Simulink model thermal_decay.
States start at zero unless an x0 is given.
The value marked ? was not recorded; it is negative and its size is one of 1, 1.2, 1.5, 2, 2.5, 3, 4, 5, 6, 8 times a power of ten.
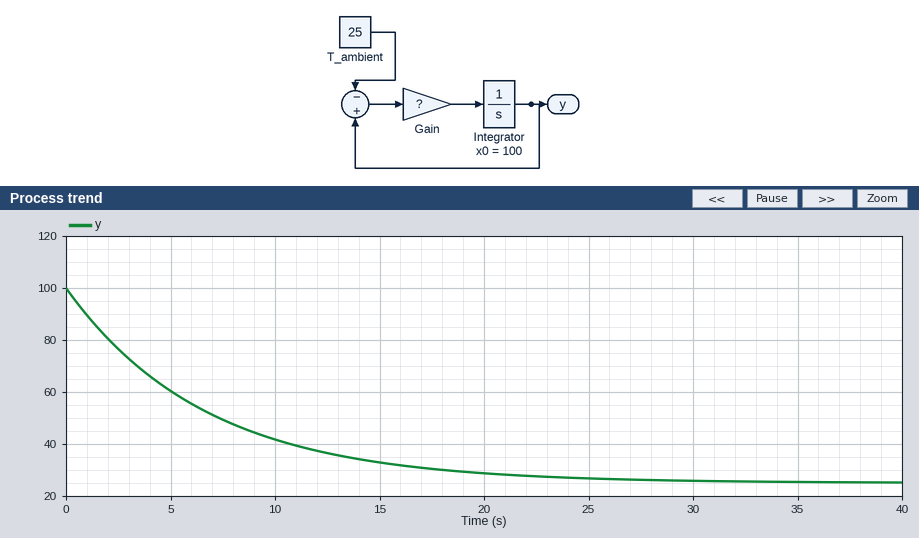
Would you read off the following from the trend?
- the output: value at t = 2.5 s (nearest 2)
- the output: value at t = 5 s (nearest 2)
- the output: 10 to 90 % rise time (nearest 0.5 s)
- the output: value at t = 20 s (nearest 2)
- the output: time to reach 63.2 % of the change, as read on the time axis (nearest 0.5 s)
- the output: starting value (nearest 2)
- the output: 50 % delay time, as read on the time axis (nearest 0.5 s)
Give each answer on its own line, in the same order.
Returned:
76
60
14.5 s
28
6.5 s
100
4.5 s
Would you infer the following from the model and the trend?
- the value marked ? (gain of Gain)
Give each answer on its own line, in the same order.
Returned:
-0.15
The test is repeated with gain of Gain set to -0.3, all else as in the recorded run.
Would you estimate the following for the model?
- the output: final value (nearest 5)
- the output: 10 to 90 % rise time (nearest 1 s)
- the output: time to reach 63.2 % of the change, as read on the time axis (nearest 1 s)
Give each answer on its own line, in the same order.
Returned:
25
7 s
3 s
